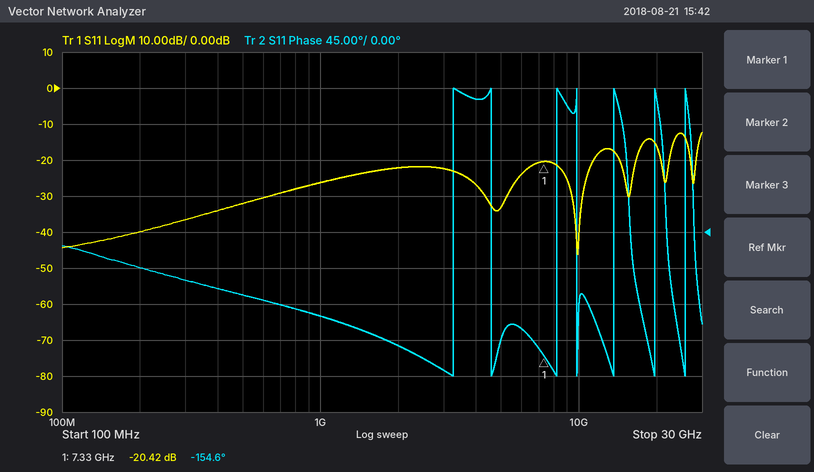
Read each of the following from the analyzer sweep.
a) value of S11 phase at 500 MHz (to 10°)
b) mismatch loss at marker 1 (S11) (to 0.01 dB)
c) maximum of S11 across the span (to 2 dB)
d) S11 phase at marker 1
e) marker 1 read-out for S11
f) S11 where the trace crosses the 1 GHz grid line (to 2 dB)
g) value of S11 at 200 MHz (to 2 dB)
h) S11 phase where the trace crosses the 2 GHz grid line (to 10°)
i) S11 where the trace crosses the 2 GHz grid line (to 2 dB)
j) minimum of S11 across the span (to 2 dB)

-80°
0.04 dB
-12 dB
-154.6°
-20.42 dB
-26 dB
-40 dB
-140°
-22 dB
-46 dB
